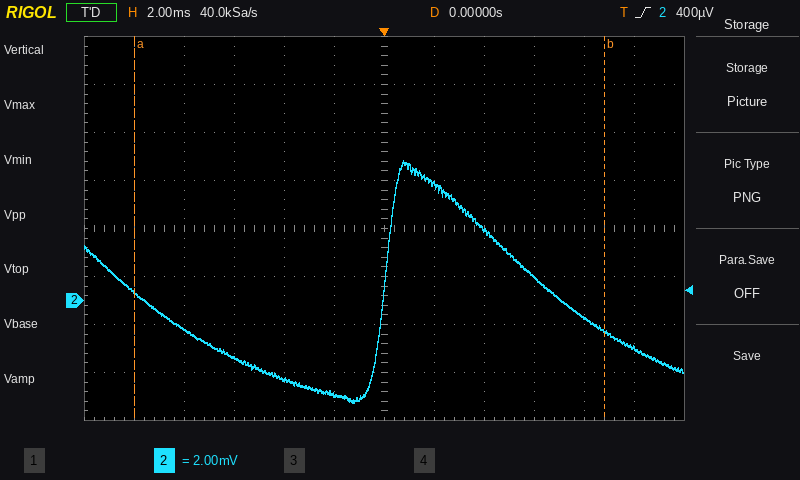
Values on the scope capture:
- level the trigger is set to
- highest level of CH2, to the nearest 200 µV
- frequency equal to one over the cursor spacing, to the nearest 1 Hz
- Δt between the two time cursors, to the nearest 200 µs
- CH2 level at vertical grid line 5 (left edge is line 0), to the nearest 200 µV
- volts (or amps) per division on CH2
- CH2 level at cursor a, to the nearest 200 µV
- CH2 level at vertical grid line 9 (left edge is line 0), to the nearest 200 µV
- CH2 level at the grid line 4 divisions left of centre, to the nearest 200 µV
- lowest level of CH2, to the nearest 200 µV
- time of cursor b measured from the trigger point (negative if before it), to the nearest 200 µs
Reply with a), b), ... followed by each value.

a) 400 µV
b) 5.8 mV
c) 53 Hz
d) 18.8 ms
e) -4.0 mV
f) 2 mV
g) 400 µV
h) 1.0 mV
i) -1.2 mV
j) -4.2 mV
k) +8.8 ms
